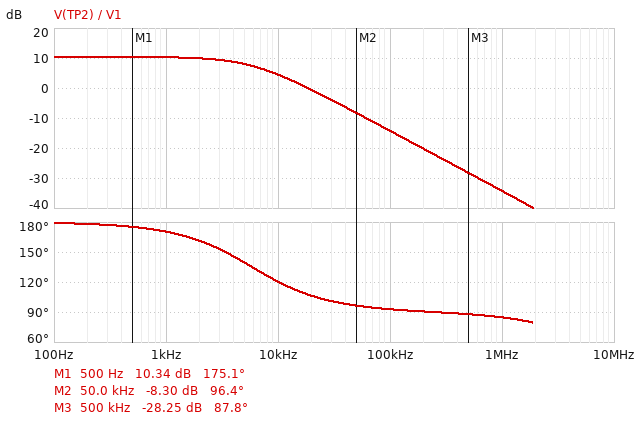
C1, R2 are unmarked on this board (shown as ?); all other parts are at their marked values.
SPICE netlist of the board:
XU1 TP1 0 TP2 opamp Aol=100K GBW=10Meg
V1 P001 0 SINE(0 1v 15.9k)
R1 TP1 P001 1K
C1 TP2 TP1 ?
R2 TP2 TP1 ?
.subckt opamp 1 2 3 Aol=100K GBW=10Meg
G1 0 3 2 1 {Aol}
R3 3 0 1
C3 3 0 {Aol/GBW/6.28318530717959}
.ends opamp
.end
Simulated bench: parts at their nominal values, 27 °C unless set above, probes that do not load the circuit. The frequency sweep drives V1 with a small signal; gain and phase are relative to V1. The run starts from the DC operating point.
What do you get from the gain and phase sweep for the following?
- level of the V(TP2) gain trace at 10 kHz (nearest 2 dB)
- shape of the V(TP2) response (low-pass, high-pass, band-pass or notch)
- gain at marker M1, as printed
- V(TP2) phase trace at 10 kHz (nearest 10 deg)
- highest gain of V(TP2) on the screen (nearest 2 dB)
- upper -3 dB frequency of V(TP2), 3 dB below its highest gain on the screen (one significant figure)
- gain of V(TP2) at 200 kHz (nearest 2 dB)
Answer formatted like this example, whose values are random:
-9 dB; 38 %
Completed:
4 dB; low-pass; 10.34 dB; 120 deg; 10 dB; 6 kHz; -20 dB
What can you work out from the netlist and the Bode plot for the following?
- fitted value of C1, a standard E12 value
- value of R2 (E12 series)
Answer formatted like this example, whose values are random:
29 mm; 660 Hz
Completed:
8.2 nF; 3.3 kΩ
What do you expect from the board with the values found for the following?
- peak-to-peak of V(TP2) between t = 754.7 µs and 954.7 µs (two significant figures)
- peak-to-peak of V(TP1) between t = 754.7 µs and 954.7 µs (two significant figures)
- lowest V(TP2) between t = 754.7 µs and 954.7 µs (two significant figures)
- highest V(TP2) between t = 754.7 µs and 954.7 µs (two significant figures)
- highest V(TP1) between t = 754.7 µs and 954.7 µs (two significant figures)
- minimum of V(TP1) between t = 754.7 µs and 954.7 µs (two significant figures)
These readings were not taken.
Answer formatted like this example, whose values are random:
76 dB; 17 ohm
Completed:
2.3 V; 3.6 mV; -1.1 V; 1.1 V; 1.8 mV; -1.8 mV
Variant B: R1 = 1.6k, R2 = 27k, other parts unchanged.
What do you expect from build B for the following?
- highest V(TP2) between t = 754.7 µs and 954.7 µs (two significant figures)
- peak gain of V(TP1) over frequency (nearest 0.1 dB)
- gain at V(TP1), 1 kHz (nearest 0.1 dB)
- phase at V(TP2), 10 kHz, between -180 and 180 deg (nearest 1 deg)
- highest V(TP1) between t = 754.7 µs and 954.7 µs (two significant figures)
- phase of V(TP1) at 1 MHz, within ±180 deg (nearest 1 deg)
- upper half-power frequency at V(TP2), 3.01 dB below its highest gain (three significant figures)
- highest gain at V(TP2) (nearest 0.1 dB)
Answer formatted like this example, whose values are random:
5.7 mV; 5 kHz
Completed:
750 mV; -58.3 dB; -60.1 dB; 94 deg; 1.2 mV; -6 deg; 718 Hz; 24.5 dB
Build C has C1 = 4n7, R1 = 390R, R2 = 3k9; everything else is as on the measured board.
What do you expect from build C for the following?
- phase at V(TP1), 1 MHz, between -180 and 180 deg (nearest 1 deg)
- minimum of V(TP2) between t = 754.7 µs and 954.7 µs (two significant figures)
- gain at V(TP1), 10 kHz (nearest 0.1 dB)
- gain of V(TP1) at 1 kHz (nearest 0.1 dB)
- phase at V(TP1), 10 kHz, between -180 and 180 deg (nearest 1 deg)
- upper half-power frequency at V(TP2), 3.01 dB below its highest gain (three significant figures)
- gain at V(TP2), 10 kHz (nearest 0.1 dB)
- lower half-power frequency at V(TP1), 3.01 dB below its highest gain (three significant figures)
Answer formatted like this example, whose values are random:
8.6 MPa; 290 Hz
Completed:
-5 deg; -4.8 V; -43.7 dB; -60.0 dB; 40 deg; 8.61 kHz; 16.3 dB; 8.59 kHz
